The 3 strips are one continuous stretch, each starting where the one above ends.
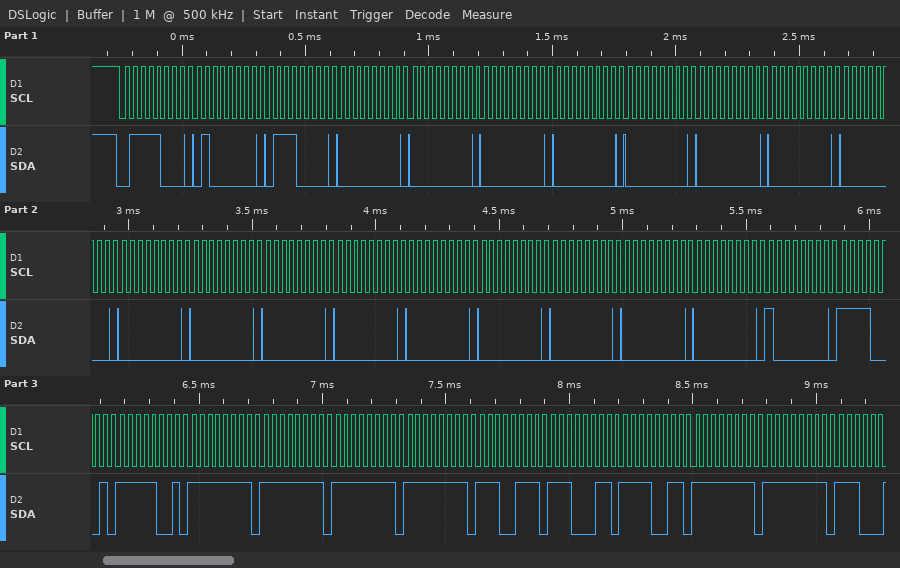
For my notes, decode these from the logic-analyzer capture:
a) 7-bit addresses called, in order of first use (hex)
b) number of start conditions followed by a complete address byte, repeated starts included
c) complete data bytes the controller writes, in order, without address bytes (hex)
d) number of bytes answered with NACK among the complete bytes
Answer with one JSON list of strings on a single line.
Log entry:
["0x3C", "1", "40 70 00 00 00 00 00 00 00 00 00 00 00 00 00 00 00 00 00 80 F1 F9 FF FF FF FF E7 E3 F3 FF FF", "0"]
